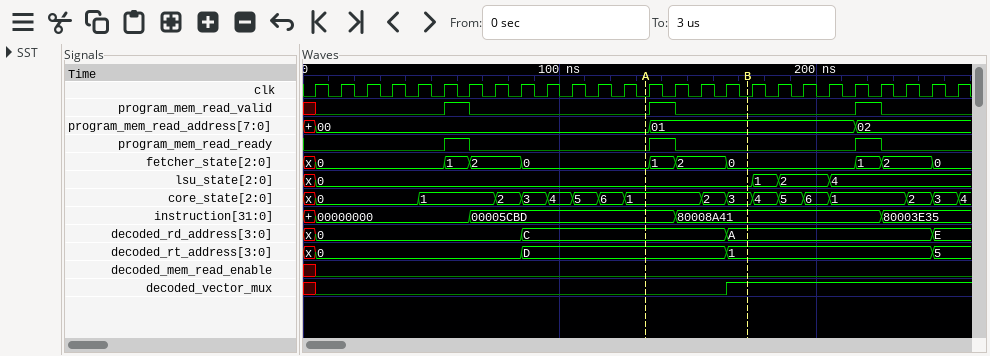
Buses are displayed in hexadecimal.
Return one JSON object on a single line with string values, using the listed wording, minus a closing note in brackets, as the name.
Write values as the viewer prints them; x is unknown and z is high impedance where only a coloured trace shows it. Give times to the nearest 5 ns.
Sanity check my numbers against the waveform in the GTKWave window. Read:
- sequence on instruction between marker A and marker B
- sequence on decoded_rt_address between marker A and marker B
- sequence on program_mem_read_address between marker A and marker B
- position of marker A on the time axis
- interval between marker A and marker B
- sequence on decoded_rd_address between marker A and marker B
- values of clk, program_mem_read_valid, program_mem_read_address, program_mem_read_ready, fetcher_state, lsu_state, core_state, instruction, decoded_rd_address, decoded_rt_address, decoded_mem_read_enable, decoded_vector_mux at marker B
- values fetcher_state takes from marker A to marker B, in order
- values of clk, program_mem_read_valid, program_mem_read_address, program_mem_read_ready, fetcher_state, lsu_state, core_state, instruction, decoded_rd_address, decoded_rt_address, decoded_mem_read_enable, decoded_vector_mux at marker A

{"sequence on instruction between marker A and marker B": "00005CBD, 80008A41", "sequence on decoded_rt_address between marker A and marker B": "D, 1", "sequence on program_mem_read_address between marker A and marker B": "00, 01", "position of marker A on the time axis": "135 ns", "interval between marker A and marker B": "40 ns", "sequence on decoded_rd_address between marker A and marker B": "C, A", "values of clk, program_mem_read_valid, program_mem_read_address, program_mem_read_ready, fetcher_state, lsu_state, core_state, instruction, decoded_rd_address, decoded_rt_address, decoded_mem_read_enable, decoded_vector_mux at marker B": "clk=0, program_mem_read_valid=0, program_mem_read_address=01, program_mem_read_ready=0, fetcher_state=0, lsu_state=0, core_state=3, instruction=80008A41, decoded_rd_address=A, decoded_rt_address=1, decoded_mem_read_enable=0, decoded_vector_mux=1", "values fetcher_state takes from marker A to marker B, in order": "0, 1, 2, 0", "values of clk, program_mem_read_valid, program_mem_read_address, program_mem_read_ready, fetcher_state, lsu_state, core_state, instruction, decoded_rd_address, decoded_rt_address, decoded_mem_read_enable, decoded_vector_mux at marker A": "clk=0, program_mem_read_valid=0, program_mem_read_address=00, program_mem_read_ready=0, fetcher_state=0, lsu_state=0, core_state=1, instruction=00005CBD, decoded_rd_address=C, decoded_rt_address=D, decoded_mem_read_enable=0, decoded_vector_mux=0"}
